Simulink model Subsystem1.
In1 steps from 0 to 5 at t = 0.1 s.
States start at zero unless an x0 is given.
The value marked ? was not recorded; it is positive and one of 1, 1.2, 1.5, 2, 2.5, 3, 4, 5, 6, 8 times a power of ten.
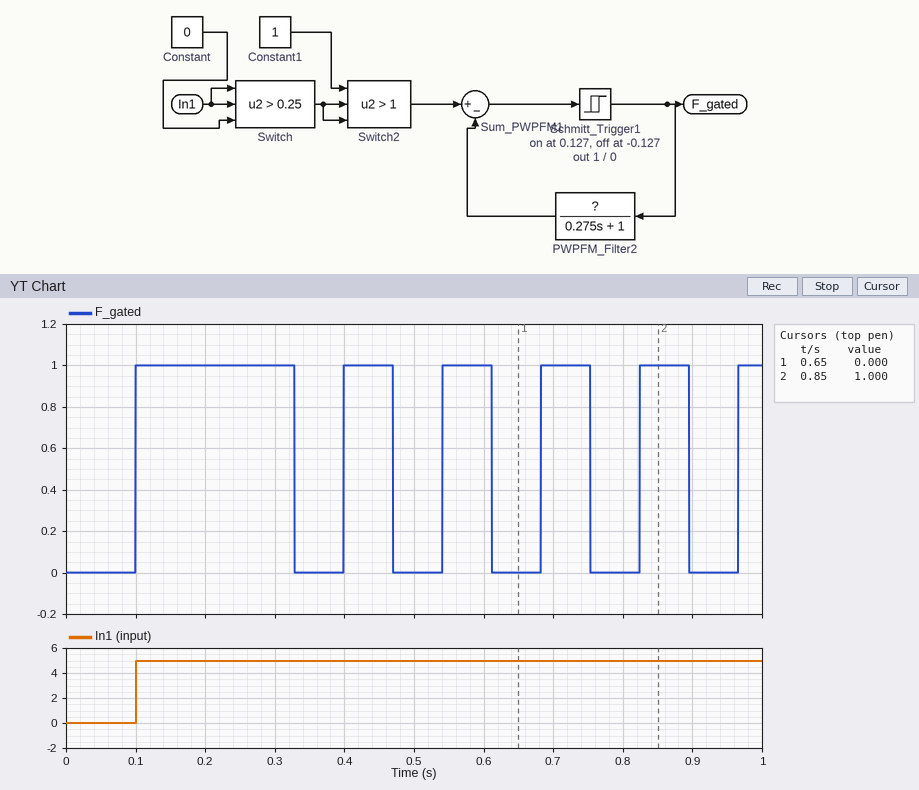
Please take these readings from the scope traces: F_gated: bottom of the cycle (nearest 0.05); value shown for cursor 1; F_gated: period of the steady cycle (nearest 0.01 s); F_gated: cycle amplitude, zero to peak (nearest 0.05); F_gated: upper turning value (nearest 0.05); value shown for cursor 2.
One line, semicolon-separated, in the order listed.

0.00; 0.000; 0.14 s; 0.50; 1.00; 1.000
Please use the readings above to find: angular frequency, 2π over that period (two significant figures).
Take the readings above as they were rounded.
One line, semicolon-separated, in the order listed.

45 rad/s
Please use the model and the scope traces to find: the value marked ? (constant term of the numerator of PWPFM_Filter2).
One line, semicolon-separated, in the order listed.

2
